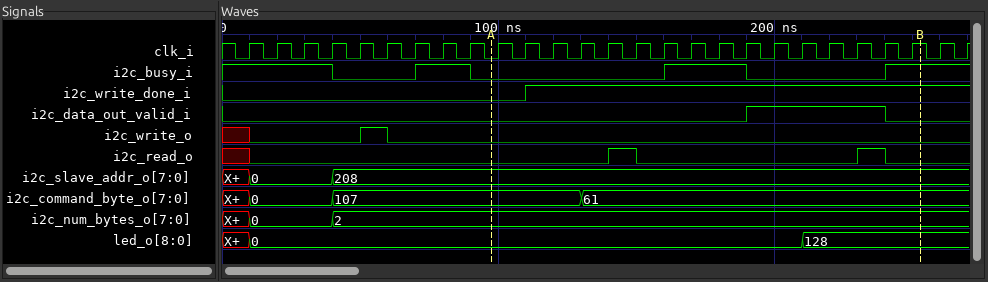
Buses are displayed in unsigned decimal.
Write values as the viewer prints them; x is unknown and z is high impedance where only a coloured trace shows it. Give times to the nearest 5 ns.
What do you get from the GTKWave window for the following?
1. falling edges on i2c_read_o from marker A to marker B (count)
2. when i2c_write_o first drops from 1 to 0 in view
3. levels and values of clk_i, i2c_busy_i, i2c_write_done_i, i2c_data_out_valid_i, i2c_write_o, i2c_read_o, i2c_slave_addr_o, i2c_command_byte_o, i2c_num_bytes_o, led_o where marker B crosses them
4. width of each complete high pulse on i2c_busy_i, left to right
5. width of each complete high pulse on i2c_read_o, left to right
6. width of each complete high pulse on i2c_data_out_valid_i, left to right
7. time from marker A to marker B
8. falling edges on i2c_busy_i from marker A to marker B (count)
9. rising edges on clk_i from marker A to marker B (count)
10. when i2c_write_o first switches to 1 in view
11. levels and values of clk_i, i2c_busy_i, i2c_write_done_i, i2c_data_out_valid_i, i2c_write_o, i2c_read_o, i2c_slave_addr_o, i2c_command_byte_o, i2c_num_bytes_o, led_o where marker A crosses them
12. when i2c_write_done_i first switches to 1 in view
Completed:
2
60 ns
clk_i=1, i2c_busy_i=1, i2c_write_done_i=1, i2c_data_out_valid_i=0, i2c_write_o=0, i2c_read_o=0, i2c_slave_addr_o=208, i2c_command_byte_o=61, i2c_num_bytes_o=2, led_o=128
20 ns, 30 ns
10 ns, 10 ns
50 ns
155 ns
1
16
50 ns
clk_i=0, i2c_busy_i=0, i2c_write_done_i=0, i2c_data_out_valid_i=0, i2c_write_o=0, i2c_read_o=0, i2c_slave_addr_o=208, i2c_command_byte_o=107, i2c_num_bytes_o=2, led_o=0
110 ns
